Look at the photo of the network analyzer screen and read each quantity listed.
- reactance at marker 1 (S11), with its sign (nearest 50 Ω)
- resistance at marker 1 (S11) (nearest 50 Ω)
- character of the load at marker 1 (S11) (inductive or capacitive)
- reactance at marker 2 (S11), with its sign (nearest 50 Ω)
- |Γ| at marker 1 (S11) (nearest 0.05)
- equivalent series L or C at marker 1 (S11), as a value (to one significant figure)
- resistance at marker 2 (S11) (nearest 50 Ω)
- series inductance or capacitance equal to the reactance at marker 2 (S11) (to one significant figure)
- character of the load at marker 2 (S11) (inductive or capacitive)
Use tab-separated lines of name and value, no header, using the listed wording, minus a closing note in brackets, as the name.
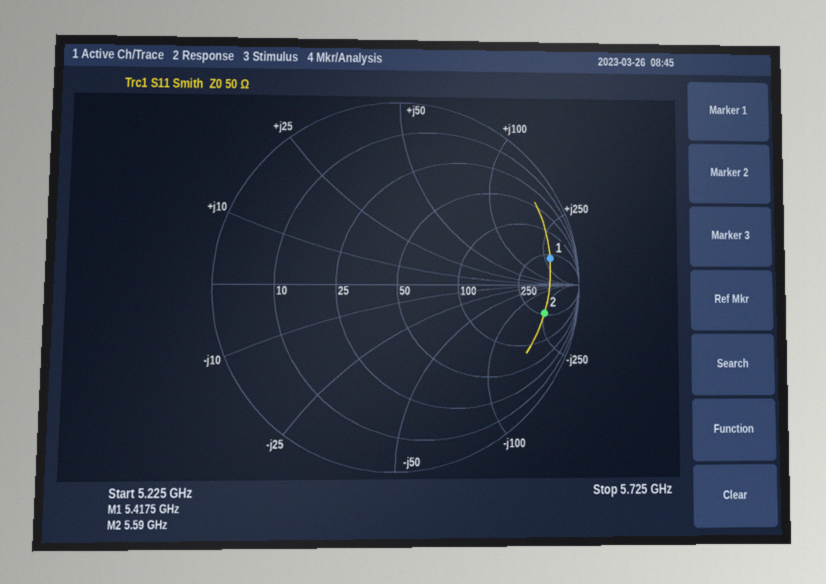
reactance at marker 1 (S11), with its sign	+300 Ω
resistance at marker 1 (S11)	300 Ω
character of the load at marker 1 (S11)	inductive
reactance at marker 2 (S11), with its sign	-250 Ω
|Γ| at marker 1 (S11)	0.85
equivalent series L or C at marker 1 (S11), as a value	9 nH
resistance at marker 2 (S11)	250 Ω
series inductance or capacitance equal to the reactance at marker 2 (S11)	100 fF
character of the load at marker 2 (S11)	capacitive
